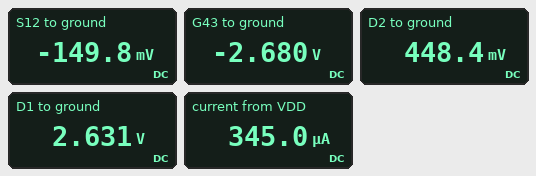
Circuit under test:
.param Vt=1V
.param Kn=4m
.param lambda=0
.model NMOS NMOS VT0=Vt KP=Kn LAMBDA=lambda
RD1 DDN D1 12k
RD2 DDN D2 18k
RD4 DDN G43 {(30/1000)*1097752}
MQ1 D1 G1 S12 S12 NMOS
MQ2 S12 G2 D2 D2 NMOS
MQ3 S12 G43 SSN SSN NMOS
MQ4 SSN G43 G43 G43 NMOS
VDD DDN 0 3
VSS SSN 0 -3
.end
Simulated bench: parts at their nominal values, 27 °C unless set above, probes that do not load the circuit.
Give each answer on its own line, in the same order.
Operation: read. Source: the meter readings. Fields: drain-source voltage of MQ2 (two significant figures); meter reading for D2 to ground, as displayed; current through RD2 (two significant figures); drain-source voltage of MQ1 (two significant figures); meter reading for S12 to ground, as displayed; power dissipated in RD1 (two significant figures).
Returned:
-600 mV
448.4 mV
140 µA
2.8 V
-149.8 mV
11 µW
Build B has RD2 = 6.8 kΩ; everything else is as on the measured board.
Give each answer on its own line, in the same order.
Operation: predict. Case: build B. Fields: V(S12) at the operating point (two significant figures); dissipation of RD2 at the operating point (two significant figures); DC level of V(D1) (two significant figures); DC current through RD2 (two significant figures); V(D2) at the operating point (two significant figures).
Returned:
1.2 V
200 µW
3.0 V
170 µA
1.8 V
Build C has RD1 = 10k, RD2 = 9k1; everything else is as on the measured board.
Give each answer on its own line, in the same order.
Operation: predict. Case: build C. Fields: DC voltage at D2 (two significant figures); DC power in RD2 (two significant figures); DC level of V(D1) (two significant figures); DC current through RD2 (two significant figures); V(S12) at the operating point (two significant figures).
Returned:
1.4 V
270 µW
3.0 V
170 µA
820 mV
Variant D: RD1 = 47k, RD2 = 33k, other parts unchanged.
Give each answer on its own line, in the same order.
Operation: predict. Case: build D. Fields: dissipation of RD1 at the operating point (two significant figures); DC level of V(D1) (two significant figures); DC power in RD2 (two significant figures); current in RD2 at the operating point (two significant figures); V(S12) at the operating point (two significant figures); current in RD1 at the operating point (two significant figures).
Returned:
240 µW
-360 mV
340 µW
100 µA
-410 mV
71 µA
